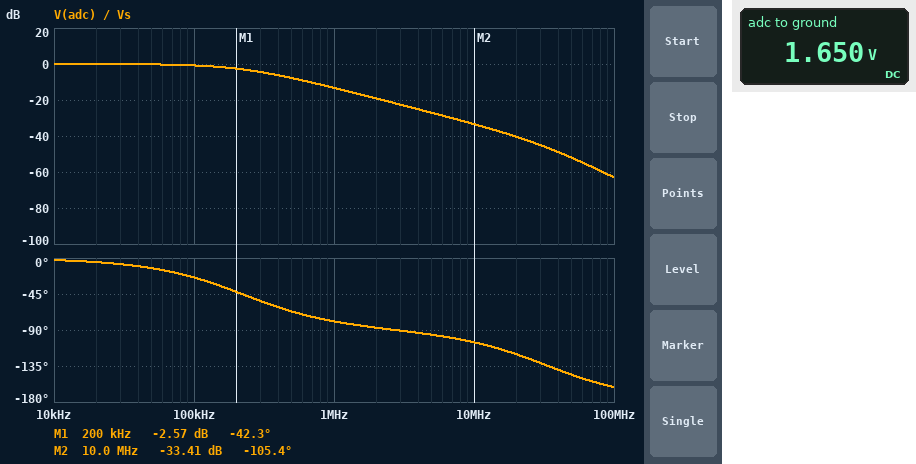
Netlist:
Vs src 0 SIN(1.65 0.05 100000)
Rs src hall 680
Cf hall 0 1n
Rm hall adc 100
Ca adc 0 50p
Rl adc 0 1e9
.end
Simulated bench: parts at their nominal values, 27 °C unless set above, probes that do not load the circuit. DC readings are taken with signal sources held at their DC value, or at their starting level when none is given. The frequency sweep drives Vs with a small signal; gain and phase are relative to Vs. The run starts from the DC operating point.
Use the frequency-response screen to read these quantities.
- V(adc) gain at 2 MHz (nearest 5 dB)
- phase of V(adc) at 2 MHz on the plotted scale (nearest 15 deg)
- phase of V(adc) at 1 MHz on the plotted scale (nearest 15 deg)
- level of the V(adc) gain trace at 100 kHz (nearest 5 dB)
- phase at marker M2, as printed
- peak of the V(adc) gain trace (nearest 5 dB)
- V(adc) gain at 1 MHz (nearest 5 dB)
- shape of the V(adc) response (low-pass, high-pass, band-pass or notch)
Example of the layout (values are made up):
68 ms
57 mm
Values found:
-20 dB
-90 deg
-75 deg
0 dB
-105.4 deg
0 dB
-15 dB
low-pass
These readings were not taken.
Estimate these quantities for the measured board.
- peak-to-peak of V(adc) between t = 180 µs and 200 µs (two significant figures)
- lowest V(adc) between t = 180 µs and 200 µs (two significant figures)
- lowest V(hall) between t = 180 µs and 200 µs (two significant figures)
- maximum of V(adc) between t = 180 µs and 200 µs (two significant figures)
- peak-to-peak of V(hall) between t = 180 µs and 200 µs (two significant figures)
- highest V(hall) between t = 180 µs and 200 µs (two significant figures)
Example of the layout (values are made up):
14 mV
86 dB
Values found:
91 mV
1.6 V
1.6 V
1.7 V
91 mV
1.7 V
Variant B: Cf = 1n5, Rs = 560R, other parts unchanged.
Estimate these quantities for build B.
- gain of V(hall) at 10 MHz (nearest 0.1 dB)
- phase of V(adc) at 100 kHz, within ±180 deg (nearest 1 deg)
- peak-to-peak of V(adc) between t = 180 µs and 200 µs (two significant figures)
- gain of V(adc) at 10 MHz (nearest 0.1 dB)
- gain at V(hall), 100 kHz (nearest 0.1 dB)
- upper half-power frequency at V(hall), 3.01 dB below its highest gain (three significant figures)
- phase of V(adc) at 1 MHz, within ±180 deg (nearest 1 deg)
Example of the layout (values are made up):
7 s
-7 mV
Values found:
-34.7 dB
-29 deg
88 mV
-35.1 dB
-1.1 dB
183 kHz
-81 deg
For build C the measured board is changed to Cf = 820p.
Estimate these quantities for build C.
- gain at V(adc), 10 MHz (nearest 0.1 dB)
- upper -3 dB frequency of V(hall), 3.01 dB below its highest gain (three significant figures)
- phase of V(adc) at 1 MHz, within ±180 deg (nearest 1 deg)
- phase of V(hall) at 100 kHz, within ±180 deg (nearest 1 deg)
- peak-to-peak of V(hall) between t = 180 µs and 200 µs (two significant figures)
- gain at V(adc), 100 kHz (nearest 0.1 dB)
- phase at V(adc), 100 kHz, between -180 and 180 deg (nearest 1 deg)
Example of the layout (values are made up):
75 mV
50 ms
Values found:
-31.8 dB
269 kHz
-77 deg
-20 deg
94 mV
-0.6 dB
-21 deg
